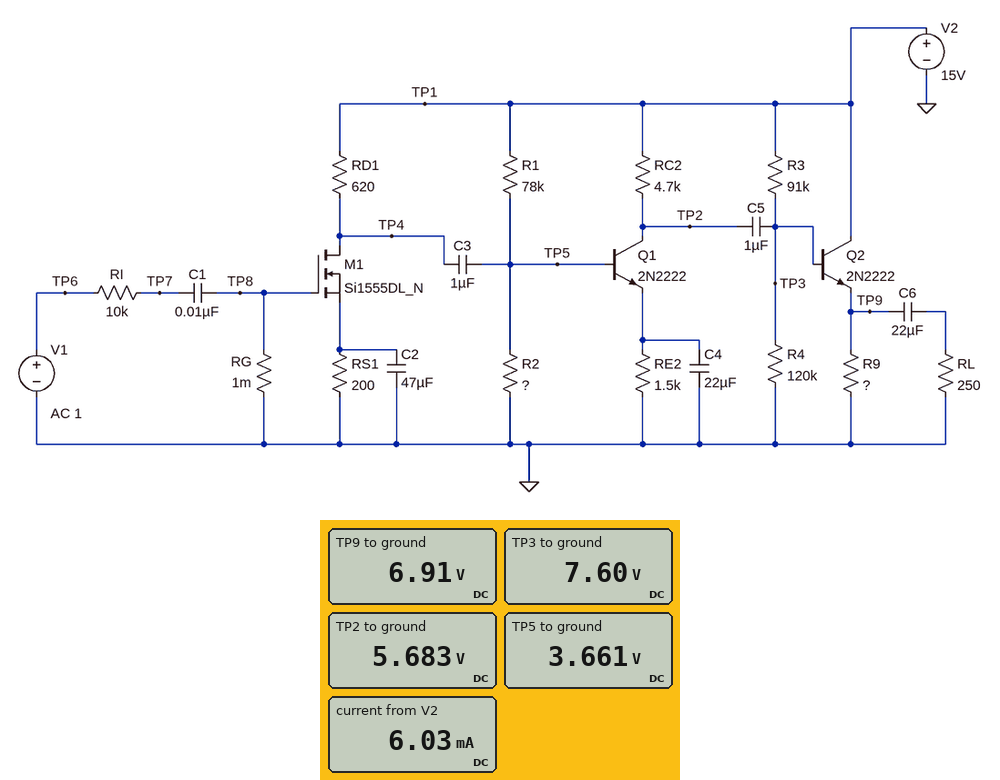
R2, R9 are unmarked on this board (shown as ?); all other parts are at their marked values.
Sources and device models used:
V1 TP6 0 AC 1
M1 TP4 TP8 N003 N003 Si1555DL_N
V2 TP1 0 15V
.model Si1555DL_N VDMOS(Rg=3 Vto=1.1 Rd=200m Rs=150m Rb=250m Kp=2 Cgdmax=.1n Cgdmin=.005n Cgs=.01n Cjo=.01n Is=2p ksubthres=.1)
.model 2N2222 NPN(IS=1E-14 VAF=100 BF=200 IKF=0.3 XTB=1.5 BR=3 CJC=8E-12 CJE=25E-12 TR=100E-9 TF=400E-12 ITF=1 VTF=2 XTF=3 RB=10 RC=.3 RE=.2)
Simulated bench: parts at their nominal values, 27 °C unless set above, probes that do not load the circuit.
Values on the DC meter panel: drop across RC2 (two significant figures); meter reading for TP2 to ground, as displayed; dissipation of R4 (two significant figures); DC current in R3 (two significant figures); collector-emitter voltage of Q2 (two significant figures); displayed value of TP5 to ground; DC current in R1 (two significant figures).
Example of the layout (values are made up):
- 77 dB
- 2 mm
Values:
- 9.3 V
- 5.683 V
- 480 µW
- 81 µA
- 8.1 V
- 3.661 V
- 150 µA
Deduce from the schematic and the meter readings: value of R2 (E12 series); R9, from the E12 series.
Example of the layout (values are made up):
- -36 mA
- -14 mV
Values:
- 27 kΩ
- 1.8 kΩ
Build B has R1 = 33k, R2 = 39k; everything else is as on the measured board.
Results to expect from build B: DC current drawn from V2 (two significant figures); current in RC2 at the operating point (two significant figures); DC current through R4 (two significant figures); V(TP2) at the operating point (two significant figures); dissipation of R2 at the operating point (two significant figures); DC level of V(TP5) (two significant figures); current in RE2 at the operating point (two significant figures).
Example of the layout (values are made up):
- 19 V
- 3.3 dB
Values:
- 6.6 mA
- 2.4 mA
- 63 µA
- 3.9 V
- 530 µW
- 4.5 V
- 2.6 mA
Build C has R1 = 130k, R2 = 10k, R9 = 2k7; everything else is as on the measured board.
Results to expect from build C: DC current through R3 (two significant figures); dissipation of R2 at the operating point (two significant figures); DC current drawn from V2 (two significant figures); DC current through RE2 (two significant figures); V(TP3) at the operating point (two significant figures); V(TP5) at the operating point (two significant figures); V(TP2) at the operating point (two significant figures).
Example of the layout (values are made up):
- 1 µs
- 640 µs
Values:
- 78 µA
- 110 µW
- 3.1 mA
- 290 µA
- 7.9 V
- 1.1 V
- 14 V
